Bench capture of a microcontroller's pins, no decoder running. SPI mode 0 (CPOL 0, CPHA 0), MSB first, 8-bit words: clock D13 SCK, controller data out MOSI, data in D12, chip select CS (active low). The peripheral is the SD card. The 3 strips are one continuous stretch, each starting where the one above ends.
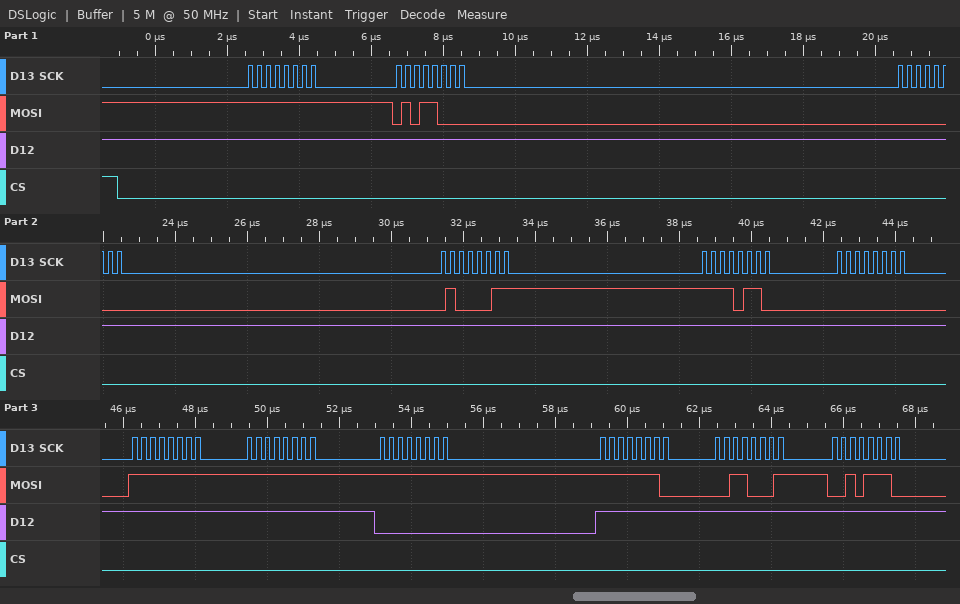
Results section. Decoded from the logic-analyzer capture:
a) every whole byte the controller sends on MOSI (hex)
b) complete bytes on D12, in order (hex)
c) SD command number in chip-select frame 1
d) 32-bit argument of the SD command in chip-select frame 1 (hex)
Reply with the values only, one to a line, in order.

FF 58 00 43 F6 00 FF FF FF FE 31 2E
FF FF FF FF FF FF FF FF 00 FF FF FF
CMD24
0x0043F600
